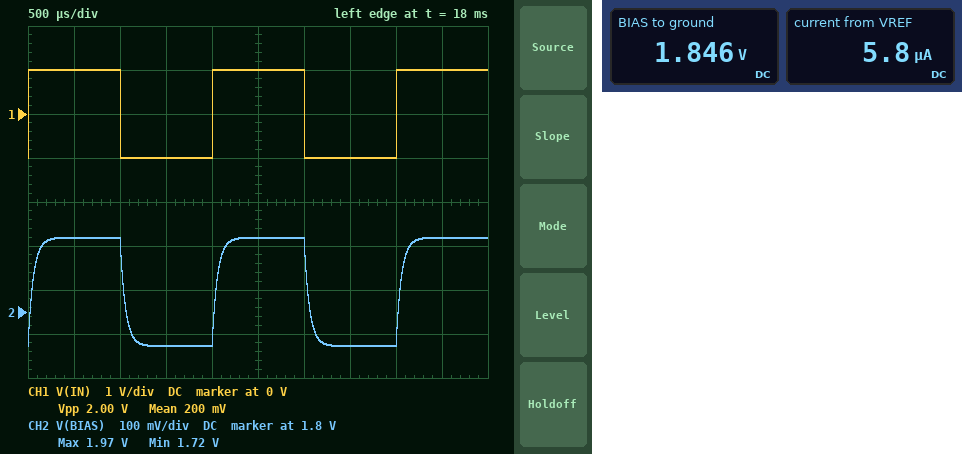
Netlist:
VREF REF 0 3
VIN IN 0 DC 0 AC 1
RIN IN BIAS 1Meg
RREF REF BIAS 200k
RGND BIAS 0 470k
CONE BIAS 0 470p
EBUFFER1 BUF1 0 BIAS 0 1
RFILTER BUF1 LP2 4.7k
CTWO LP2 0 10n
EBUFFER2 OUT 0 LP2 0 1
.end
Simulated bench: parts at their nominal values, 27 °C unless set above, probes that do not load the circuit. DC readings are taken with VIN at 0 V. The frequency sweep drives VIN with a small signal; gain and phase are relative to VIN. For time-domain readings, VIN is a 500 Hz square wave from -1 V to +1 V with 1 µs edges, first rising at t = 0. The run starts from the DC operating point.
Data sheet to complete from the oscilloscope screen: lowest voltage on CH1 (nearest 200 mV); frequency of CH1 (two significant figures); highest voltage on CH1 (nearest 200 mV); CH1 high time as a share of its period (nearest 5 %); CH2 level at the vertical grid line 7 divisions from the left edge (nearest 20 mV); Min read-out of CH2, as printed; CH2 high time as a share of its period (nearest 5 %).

-1.0 V
500 Hz
1.0 V
50 %
1.72 V
1.72 V
50 %
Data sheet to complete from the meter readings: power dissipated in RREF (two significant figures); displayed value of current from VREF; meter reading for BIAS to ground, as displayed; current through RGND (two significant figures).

6.7 µW
5.8 µA
1.846 V
3.9 µA
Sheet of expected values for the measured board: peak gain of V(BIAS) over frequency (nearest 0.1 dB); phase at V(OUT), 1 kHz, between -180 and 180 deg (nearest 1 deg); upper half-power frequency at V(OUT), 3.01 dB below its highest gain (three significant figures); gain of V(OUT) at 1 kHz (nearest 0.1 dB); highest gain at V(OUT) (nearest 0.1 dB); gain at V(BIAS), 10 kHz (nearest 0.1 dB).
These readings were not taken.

-18.2 dB
-36 deg
1.95 kHz
-19.1 dB
-18.2 dB
-29.7 dB
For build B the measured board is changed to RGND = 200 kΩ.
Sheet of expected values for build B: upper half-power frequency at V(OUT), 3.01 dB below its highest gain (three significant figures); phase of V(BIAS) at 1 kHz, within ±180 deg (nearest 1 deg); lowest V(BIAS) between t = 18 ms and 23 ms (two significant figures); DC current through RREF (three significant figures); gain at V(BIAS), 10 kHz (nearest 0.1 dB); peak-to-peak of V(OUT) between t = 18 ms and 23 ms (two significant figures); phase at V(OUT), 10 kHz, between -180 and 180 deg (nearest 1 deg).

2.28 kHz
-15 deg
1.3 V
8.18 µA
-30.0 dB
180 mV
-141 deg
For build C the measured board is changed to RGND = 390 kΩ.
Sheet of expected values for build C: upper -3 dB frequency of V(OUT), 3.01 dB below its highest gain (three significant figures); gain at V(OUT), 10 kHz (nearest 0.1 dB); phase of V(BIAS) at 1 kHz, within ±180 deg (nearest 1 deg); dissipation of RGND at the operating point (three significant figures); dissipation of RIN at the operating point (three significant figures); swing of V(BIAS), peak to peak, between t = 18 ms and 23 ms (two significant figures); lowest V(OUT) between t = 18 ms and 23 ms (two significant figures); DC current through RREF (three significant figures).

2.01 kHz
-39.6 dB
-19 deg
7.87 µW
3.07 µW
230 mV
1.6 V
6.24 µA
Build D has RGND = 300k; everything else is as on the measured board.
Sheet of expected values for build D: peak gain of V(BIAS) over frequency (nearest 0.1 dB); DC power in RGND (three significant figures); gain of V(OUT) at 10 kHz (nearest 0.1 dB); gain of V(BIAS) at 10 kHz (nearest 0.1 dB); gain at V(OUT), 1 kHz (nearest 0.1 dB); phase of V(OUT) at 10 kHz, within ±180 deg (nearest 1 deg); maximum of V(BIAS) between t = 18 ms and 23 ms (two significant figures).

-19.4 dB
8.61 µW
-39.7 dB
-29.8 dB
-20.2 dB
-144 deg
1.7 V
